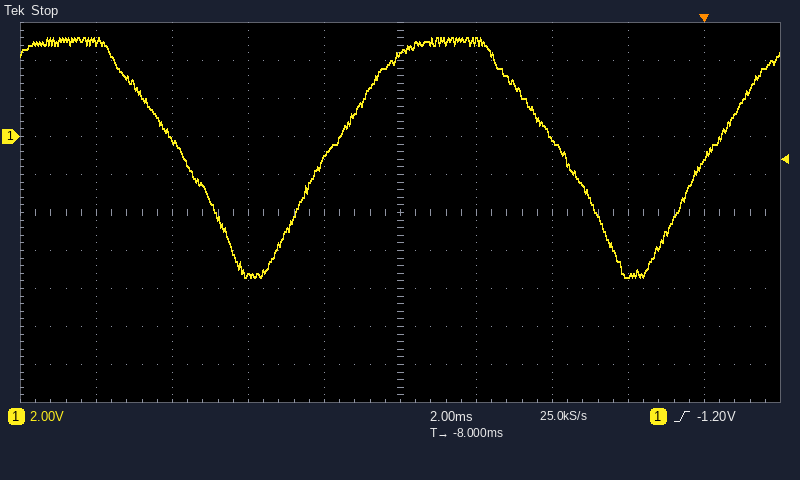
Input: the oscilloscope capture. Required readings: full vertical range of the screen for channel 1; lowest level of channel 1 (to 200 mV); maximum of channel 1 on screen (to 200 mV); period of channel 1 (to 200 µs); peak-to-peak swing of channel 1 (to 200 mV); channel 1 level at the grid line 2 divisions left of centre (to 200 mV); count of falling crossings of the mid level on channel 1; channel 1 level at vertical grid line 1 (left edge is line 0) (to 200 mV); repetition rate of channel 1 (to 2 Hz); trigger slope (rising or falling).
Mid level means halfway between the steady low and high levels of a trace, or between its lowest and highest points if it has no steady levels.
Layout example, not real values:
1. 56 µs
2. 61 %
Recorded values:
1. 20 V
2. -7.4 V
3. 5.2 V
4. 10.0 ms
5. 12.6 V
6. -7.2 V
7. 2
8. 5.0 V
9. 100 Hz
10. rising
